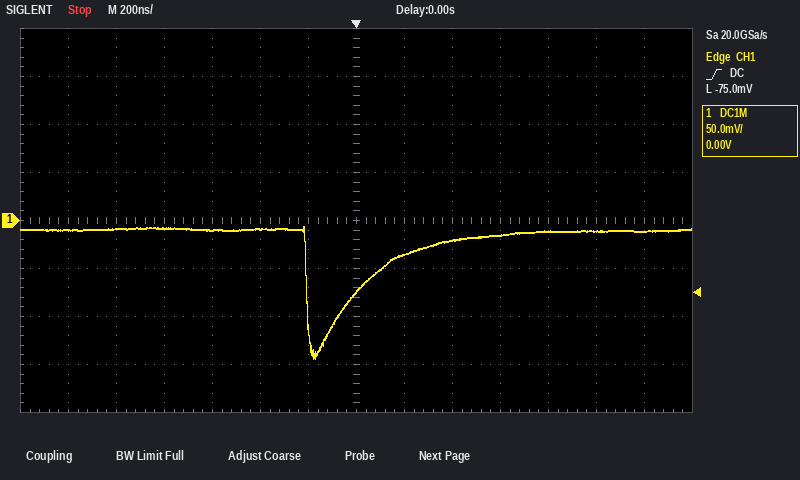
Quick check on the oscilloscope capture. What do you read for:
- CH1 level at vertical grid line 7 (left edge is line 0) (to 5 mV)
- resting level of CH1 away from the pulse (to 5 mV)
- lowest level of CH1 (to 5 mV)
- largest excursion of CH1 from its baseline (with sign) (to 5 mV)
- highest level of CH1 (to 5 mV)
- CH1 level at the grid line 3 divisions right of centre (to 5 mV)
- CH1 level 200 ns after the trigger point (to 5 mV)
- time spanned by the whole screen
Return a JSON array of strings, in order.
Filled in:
["-75 mV", "-10 mV", "-145 mV", "-135 mV", "-5 mV", "-15 mV", "-35 mV", "2.8 µs"]
